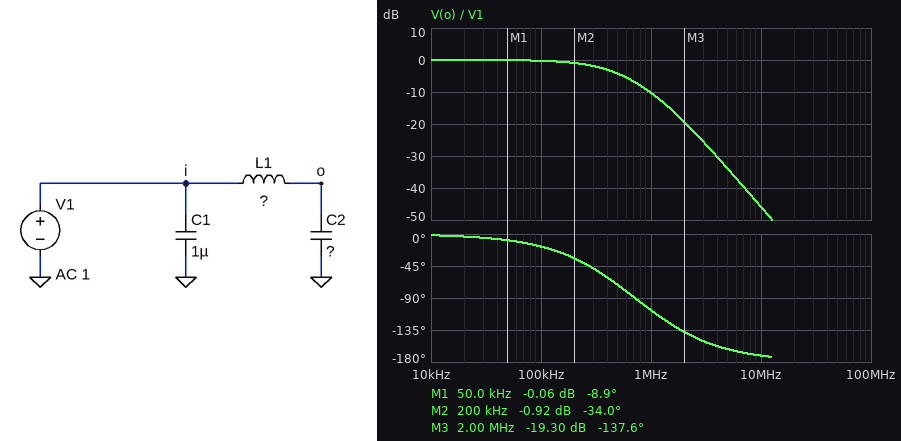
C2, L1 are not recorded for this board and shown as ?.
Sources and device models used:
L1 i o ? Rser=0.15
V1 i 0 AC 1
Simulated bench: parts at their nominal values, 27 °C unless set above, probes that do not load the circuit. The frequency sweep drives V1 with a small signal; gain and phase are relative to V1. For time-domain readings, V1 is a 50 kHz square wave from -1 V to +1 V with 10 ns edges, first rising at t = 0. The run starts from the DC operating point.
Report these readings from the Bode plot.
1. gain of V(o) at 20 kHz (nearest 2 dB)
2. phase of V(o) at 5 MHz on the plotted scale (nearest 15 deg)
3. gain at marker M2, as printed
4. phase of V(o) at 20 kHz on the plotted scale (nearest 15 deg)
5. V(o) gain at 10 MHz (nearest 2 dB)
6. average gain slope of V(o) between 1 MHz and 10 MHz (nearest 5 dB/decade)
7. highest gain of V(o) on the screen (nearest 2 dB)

0 dB
-165 deg
-0.92 dB
0 deg
-46 dB
-35 dB/decade
0 dB
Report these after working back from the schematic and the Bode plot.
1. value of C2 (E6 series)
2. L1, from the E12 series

3.3 µF
15 nH
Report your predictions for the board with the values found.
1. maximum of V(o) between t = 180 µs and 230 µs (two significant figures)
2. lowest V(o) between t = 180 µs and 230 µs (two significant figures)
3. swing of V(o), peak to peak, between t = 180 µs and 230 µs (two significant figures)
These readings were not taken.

1.0 V
-1.0 V
2.0 V
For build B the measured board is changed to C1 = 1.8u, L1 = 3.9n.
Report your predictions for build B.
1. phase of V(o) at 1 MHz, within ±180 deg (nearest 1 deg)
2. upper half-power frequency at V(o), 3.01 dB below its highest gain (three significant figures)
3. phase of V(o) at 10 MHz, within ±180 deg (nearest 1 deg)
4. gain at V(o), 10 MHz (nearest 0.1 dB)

-81 deg
339 kHz
-148 deg
-35.4 dB
